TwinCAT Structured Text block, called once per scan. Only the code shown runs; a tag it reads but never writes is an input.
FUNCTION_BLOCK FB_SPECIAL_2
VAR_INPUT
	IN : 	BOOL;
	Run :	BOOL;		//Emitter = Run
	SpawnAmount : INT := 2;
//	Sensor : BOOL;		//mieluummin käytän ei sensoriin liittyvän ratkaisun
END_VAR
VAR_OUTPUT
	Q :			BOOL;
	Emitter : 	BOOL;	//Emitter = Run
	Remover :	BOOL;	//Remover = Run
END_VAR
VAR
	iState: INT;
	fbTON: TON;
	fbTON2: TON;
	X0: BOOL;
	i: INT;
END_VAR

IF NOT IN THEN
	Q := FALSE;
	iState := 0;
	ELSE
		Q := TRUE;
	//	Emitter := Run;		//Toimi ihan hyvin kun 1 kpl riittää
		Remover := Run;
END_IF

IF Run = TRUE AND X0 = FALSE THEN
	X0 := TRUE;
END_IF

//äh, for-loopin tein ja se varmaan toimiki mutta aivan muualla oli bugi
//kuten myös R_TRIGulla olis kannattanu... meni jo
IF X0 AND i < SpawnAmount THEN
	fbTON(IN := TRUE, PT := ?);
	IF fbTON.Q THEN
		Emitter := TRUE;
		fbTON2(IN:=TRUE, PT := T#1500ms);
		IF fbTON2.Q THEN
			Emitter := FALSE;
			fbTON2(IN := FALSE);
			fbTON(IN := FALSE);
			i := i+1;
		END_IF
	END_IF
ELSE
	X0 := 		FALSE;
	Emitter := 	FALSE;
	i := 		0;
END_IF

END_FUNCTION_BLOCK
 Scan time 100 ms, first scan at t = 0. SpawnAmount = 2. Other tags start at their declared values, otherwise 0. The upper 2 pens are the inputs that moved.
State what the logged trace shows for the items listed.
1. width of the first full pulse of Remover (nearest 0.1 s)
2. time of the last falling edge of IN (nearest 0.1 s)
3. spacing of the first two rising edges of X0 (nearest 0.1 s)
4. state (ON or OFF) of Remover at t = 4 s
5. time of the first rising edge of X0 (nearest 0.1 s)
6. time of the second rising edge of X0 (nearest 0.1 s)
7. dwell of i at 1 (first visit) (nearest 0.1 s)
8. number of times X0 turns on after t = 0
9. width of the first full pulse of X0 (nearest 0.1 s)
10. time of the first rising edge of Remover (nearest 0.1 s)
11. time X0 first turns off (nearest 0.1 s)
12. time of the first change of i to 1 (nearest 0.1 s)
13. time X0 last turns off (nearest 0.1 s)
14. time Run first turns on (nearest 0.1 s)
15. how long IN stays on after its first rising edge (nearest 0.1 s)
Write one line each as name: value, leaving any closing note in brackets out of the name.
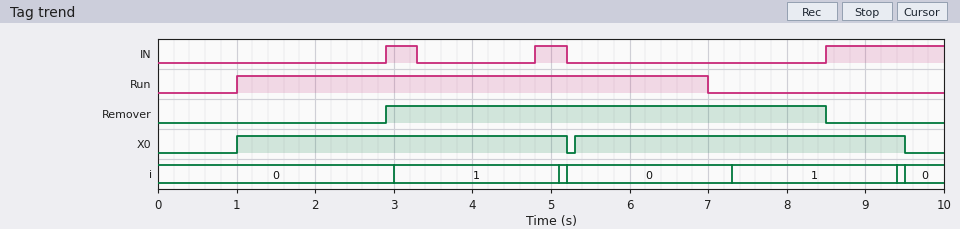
width of the first full pulse of Remover: 5.6 s
time of the last falling edge of IN: 5.2 s
spacing of the first two rising edges of X0: 4.3 s
state (ON or OFF) of Remover at t = 4 s: ON
time of the first rising edge of X0: 1.0 s
time of the second rising edge of X0: 5.3 s
dwell of i at 1 (first visit): 2.1 s
number of times X0 turns on after t = 0: 2
width of the first full pulse of X0: 4.2 s
time of the first rising edge of Remover: 2.9 s
time X0 first turns off: 5.2 s
time of the first change of i to 1: 3.0 s
time X0 last turns off: 9.5 s
time Run first turns on: 1.0 s
how long IN stays on after its first rising edge: 0.4 s
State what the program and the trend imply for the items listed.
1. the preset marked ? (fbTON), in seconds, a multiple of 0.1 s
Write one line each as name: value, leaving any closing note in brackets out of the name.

the preset marked ? (fbTON), in seconds, a multiple of 0.1 s: 0.5 s
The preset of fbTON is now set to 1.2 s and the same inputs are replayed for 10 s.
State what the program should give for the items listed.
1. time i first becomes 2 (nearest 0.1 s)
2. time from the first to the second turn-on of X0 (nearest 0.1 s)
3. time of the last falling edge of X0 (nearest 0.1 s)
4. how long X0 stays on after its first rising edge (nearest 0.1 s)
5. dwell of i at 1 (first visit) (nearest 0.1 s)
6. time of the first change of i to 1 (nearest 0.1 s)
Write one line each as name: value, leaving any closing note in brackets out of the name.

time i first becomes 2: 6.5 s
time from the first to the second turn-on of X0: 5.7 s
time of the last falling edge of X0: 6.6 s
how long X0 stays on after its first rising edge: 5.6 s
dwell of i at 1 (first visit): 2.8 s
time of the first change of i to 1: 3.7 s
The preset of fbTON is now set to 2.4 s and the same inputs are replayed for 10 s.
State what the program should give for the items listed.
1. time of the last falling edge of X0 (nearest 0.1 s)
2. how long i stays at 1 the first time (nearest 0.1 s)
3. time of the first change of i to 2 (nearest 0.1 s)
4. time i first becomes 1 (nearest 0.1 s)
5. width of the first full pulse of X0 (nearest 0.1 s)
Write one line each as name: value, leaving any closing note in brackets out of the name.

time of the last falling edge of X0: 9.0 s
how long i stays at 1 the first time: 4.0 s
time of the first change of i to 2: 8.9 s
time i first becomes 1: 4.9 s
width of the first full pulse of X0: 8.0 s
